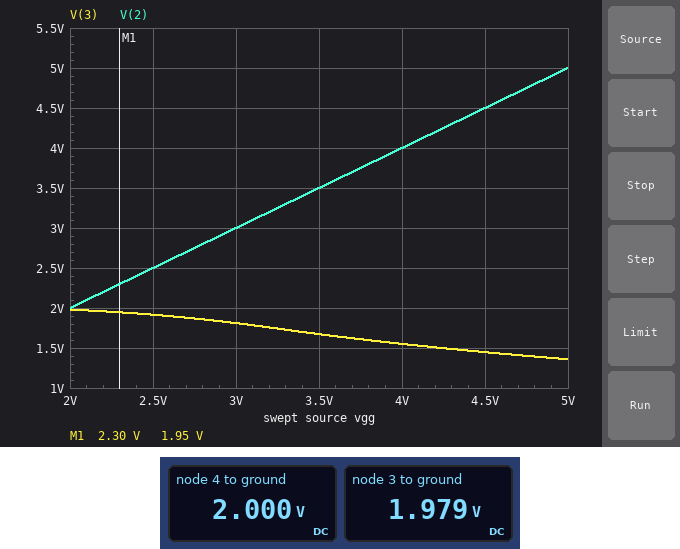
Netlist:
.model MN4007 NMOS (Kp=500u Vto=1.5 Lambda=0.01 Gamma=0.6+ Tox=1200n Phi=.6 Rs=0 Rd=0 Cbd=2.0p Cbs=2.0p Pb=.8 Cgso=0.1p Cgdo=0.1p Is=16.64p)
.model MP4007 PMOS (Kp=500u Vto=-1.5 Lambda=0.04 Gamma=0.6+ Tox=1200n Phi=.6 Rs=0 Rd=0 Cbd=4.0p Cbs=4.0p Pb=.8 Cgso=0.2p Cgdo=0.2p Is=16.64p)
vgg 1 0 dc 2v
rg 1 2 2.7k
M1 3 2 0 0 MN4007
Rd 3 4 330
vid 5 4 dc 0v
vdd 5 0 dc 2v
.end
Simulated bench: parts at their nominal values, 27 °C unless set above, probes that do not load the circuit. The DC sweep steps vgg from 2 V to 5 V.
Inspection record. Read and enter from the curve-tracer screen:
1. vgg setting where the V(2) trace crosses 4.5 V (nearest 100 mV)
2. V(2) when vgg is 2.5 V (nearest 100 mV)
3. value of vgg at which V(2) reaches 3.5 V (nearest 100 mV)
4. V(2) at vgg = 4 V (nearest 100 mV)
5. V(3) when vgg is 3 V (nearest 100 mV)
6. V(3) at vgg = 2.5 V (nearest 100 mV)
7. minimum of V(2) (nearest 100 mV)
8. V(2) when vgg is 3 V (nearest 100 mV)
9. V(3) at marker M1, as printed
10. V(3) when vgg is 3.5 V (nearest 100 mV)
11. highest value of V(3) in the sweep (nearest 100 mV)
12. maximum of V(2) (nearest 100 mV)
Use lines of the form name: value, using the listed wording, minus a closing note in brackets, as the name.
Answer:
vgg setting where the V(2) trace crosses 4.5 V: 4.5 V
V(2) when vgg is 2.5 V: 2.5 V
value of vgg at which V(2) reaches 3.5 V: 3.5 V
V(2) at vgg = 4 V: 4.0 V
V(3) when vgg is 3 V: 1.8 V
V(3) at vgg = 2.5 V: 1.9 V
minimum of V(2): 2.0 V
V(2) when vgg is 3 V: 3.0 V
V(3) at marker M1, as printed: 1.95 V
V(3) when vgg is 3.5 V: 1.7 V
highest value of V(3) in the sweep: 2.0 V
maximum of V(2): 5.0 V
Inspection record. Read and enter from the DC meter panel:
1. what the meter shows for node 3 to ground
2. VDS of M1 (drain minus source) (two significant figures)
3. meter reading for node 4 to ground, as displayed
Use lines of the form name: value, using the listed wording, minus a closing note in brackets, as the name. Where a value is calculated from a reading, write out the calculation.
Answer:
what the meter shows for node 3 to ground: 1.979 V
VDS of M1 (drain minus source): 1.979 V = 2.0 V
meter reading for node 4 to ground, as displayed: 2.000 V
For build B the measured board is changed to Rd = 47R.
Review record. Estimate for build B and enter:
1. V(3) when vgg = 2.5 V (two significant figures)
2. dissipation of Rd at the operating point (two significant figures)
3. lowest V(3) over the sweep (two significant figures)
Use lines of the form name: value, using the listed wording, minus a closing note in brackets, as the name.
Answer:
V(3) when vgg = 2.5 V: 2.0 V
dissipation of Rd at the operating point: 190 nW
lowest V(3) over the sweep: 1.9 V
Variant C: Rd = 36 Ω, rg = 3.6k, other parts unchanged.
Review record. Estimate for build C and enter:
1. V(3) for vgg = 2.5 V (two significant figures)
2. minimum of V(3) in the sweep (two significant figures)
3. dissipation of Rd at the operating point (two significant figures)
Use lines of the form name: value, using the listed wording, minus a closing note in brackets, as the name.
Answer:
V(3) for vgg = 2.5 V: 2.0 V
minimum of V(3) in the sweep: 1.9 V
dissipation of Rd at the operating point: 150 nW
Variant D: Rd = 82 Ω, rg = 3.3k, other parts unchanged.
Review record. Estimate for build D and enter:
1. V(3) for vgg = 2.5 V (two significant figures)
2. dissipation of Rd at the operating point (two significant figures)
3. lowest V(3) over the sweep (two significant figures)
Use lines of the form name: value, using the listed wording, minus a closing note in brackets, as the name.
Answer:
V(3) for vgg = 2.5 V: 2.0 V
dissipation of Rd at the operating point: 330 nW
lowest V(3) over the sweep: 1.8 V
